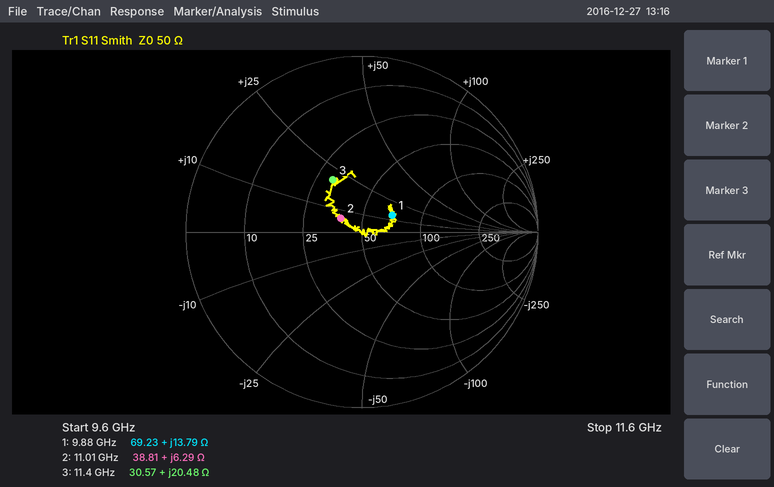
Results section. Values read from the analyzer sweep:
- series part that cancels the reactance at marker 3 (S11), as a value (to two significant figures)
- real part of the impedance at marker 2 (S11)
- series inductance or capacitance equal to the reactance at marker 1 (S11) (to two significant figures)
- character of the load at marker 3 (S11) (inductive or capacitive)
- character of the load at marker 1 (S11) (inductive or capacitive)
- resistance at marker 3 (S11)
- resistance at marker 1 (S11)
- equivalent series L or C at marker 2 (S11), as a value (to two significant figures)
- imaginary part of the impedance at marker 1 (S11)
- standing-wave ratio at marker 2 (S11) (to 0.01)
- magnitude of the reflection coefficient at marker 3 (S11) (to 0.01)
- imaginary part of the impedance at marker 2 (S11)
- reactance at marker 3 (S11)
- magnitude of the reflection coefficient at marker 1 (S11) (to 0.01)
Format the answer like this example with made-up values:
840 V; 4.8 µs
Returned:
680 fF; 38.81 Ω; 220 pH; inductive; inductive; 30.57 Ω; 69.23 Ω; 91 pH; +13.79 Ω; 1.34; 0.34; +6.29 Ω; +20.48 Ω; 0.20
